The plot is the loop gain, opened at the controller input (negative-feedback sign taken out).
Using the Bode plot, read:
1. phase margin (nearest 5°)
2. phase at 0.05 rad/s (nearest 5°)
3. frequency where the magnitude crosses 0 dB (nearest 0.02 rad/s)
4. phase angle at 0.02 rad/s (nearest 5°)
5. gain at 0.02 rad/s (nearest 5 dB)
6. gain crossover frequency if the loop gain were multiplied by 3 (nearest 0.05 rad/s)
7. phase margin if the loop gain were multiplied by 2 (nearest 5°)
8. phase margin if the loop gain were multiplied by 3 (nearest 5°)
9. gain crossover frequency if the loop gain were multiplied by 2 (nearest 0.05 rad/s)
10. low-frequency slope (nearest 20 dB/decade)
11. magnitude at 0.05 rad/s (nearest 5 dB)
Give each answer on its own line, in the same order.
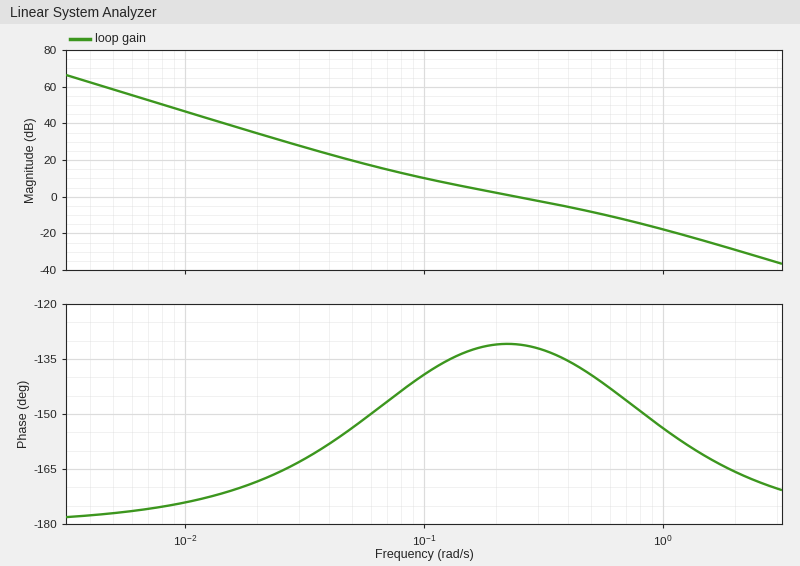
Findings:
50°
-155°
0.24 rad/s
-170°
35 dB
0.55 rad/s
45°
40°
0.40 rad/s
-40 dB/decade
20 dB
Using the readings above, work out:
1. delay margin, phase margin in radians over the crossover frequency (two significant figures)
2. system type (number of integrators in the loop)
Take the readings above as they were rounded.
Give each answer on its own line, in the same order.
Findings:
3.6 s
2
